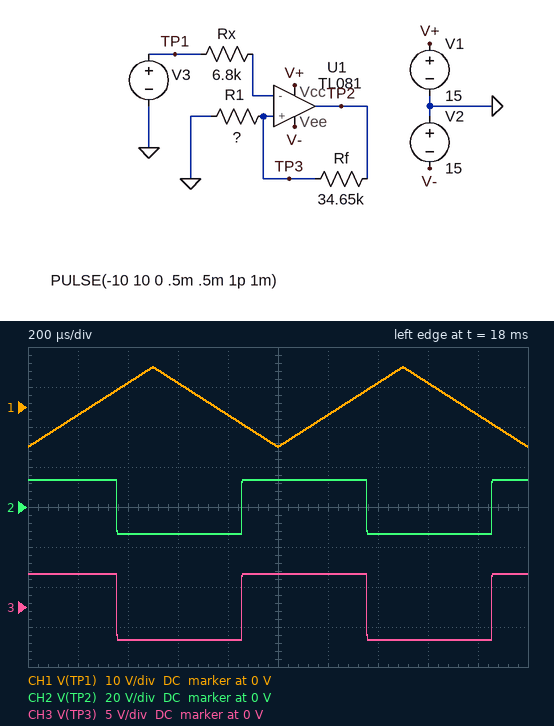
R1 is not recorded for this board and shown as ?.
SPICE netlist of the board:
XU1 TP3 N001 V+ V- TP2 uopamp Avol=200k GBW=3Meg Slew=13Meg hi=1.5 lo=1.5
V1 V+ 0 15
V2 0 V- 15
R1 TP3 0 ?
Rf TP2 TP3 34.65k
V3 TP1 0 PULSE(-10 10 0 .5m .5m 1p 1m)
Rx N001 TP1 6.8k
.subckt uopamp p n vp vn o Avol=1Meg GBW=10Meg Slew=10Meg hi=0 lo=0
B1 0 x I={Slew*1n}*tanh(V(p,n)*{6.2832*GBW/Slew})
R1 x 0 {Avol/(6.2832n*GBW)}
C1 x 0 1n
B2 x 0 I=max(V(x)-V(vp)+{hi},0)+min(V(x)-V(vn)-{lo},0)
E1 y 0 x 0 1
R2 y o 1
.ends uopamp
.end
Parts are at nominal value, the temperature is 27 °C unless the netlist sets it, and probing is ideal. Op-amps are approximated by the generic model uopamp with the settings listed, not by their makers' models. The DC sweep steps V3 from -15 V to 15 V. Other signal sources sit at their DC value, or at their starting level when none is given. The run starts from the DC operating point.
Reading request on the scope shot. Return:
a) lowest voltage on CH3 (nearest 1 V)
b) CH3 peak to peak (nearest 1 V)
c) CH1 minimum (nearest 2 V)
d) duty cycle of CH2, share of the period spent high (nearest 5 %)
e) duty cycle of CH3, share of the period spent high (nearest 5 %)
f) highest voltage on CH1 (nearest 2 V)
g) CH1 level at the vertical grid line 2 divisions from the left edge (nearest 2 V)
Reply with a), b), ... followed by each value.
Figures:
a) -4 V
b) 8 V
c) -10 V
d) 50 %
e) 50 %
f) 10 V
g) 6 V
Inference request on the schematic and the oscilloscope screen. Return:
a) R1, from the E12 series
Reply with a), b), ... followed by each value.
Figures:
a) 15 kΩ
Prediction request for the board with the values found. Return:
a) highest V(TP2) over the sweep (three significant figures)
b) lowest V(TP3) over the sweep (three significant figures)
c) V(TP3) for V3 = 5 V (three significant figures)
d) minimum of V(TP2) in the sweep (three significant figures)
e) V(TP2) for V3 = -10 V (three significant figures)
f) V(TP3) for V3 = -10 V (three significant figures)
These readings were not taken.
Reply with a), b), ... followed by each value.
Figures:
a) 13.5 V
b) -4.08 V
c) -4.08 V
d) -13.5 V
e) 13.5 V
f) 4.08 V
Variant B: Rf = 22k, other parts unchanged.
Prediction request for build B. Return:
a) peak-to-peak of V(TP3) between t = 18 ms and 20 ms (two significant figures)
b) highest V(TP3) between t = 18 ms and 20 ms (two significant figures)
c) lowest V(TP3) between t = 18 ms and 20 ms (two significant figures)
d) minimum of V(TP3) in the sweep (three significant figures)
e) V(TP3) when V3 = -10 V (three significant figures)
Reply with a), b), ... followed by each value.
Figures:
a) 11 V
b) 5.5 V
c) -5.5 V
d) -5.48 V
e) 5.48 V
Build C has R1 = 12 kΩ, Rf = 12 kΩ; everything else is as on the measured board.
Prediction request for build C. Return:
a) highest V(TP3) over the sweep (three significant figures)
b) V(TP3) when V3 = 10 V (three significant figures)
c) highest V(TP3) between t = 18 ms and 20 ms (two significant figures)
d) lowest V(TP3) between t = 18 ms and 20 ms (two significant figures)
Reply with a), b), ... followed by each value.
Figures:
a) 6.76 V
b) -6.76 V
c) 6.8 V
d) -6.8 V
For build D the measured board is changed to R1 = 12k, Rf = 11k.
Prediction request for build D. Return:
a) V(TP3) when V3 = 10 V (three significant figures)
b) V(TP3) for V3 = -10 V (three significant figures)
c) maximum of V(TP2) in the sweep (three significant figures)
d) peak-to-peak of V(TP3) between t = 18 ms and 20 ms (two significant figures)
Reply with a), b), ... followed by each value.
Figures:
a) -7.05 V
b) 7.05 V
c) 13.5 V
d) 14 V
